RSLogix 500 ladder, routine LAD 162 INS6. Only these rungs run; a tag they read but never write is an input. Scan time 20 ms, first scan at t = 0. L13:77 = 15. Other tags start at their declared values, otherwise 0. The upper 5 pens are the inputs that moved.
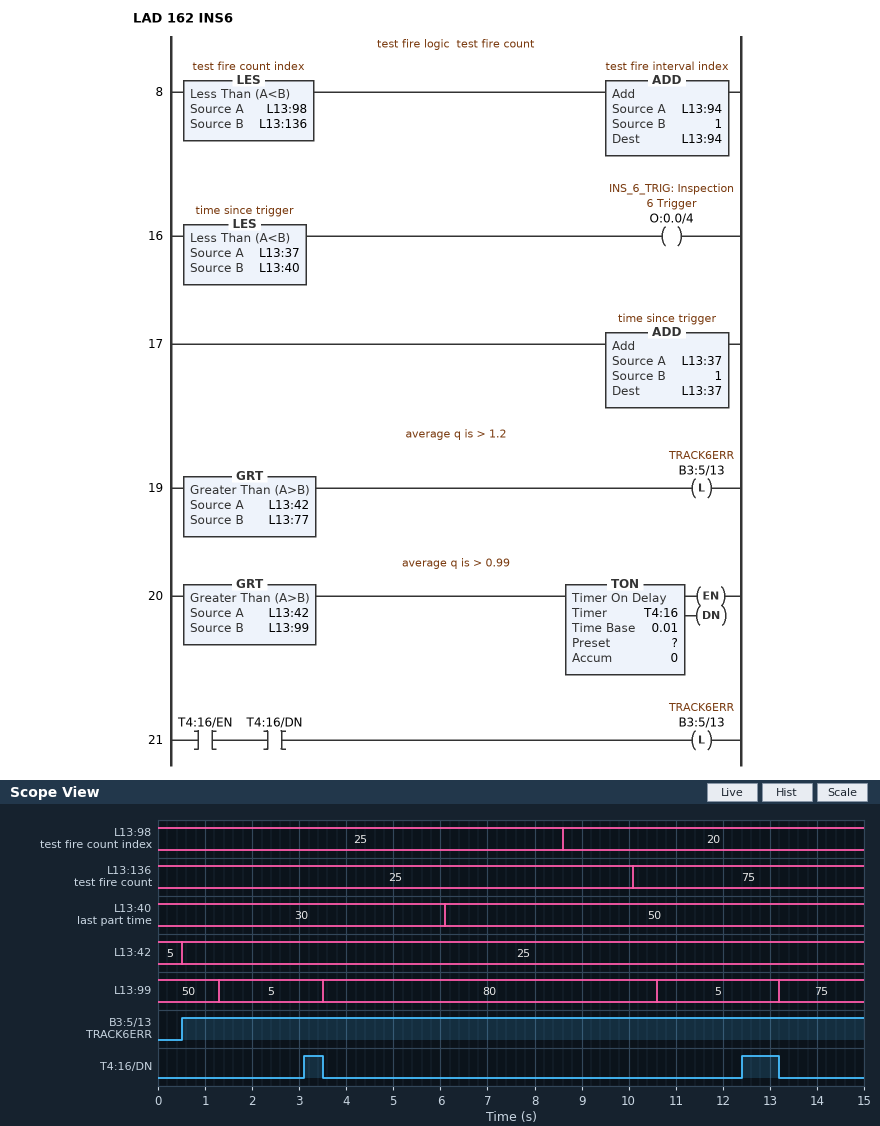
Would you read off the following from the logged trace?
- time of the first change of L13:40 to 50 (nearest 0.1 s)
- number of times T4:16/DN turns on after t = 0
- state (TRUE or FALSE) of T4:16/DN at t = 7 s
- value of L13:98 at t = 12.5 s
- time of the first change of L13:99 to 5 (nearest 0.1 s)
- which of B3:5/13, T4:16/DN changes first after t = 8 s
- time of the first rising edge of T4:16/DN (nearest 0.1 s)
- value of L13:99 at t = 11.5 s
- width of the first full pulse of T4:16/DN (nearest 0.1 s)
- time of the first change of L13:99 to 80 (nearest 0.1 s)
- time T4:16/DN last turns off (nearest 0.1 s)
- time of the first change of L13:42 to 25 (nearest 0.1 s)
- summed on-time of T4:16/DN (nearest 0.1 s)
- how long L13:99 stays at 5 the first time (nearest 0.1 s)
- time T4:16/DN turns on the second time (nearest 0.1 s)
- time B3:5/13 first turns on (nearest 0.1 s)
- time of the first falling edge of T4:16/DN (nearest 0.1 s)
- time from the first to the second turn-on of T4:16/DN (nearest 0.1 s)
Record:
6.1 s
2
FALSE
20
1.3 s
T4:16/DN
3.1 s
5
0.4 s
3.5 s
13.2 s
0.5 s
1.2 s
2.2 s
12.4 s
0.5 s
3.5 s
9.3 s
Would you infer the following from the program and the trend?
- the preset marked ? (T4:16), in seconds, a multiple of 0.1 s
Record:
1.8 s
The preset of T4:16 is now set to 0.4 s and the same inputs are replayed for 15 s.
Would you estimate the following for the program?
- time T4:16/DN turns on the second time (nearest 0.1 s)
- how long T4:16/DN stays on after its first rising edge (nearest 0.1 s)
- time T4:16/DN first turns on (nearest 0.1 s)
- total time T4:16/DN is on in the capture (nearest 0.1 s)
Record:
11.0 s
1.8 s
1.7 s
4.0 s
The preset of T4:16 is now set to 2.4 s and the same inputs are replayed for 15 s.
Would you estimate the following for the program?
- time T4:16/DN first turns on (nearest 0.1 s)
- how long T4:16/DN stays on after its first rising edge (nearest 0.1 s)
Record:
13.0 s
0.2 s
